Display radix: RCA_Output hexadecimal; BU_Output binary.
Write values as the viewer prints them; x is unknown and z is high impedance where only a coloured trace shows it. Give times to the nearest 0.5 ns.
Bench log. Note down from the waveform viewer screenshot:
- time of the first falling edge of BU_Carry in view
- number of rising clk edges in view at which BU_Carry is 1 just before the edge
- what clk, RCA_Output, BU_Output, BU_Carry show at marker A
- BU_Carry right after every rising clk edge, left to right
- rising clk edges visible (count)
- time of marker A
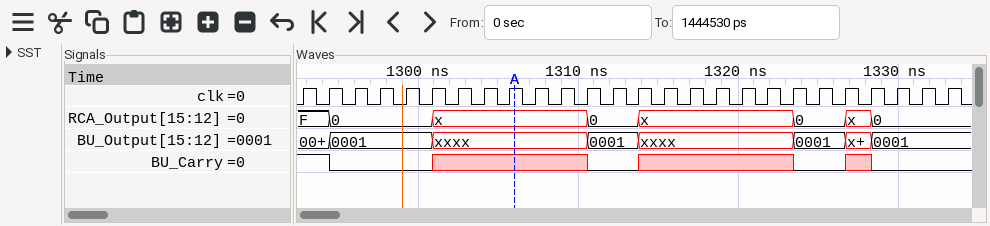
1294.5 ns
2
clk=1, RCA_Output=x, BU_Output=xxxx, BU_Carry=x
1 0 0 0 0 x x x x x x 0 0 x x x x x x 0 0 x 0 0 0 0
26
1306 ns
